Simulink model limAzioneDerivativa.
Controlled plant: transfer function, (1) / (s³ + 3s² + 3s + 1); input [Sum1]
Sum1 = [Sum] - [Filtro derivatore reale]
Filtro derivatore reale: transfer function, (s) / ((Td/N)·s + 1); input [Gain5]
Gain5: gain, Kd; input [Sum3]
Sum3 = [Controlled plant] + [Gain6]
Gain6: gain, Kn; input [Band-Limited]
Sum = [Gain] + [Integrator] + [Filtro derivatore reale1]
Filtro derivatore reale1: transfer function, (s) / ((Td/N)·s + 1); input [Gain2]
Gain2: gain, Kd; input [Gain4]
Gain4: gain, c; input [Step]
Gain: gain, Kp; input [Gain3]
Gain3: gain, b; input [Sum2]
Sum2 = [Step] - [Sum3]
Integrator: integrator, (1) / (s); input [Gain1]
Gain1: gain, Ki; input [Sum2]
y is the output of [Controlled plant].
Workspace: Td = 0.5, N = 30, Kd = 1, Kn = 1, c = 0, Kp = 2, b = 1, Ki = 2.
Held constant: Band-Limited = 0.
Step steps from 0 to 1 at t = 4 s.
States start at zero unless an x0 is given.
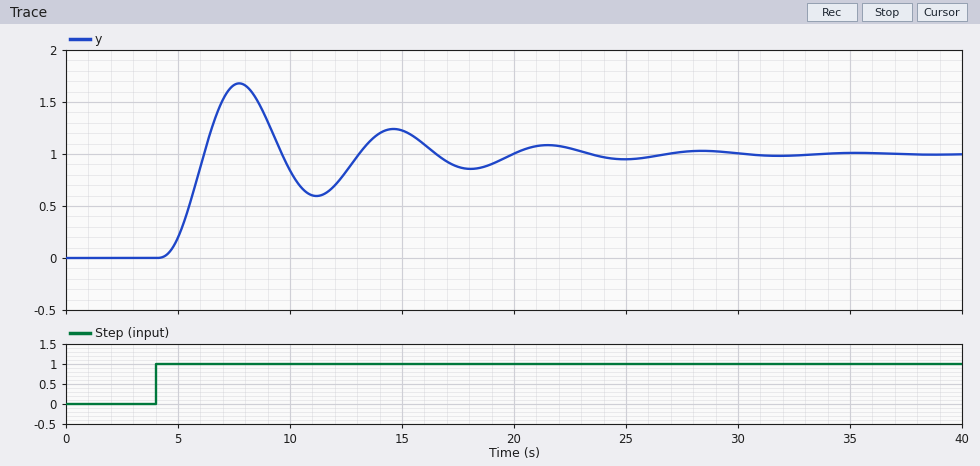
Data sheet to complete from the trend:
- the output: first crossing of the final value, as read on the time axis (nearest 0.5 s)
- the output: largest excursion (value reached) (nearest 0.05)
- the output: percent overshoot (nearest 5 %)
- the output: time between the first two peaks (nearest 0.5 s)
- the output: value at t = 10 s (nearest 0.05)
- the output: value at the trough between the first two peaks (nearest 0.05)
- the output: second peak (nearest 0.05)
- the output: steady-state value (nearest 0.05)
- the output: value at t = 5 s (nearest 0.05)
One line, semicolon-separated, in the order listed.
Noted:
6.0 s; 1.70; 70 %; 7.0 s; 0.85; 0.60; 1.25; 1.00; 0.20
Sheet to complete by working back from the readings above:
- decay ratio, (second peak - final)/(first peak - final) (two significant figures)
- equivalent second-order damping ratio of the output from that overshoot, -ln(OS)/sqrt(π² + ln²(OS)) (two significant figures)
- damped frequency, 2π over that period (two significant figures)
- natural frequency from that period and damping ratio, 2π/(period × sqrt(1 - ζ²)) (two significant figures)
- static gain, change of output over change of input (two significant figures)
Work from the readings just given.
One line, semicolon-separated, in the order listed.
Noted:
0.36; 0.11; 0.90 rad/s; 0.90 rad/s; 1.0
